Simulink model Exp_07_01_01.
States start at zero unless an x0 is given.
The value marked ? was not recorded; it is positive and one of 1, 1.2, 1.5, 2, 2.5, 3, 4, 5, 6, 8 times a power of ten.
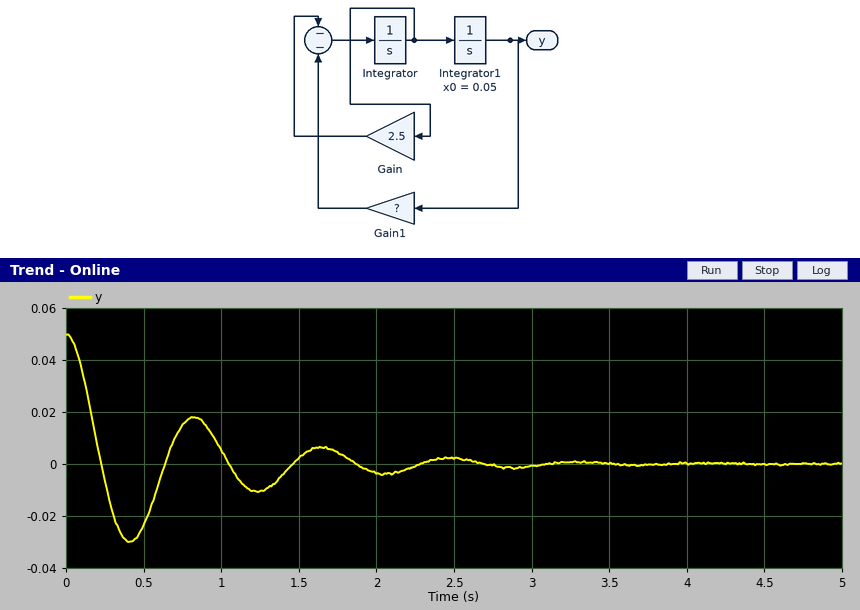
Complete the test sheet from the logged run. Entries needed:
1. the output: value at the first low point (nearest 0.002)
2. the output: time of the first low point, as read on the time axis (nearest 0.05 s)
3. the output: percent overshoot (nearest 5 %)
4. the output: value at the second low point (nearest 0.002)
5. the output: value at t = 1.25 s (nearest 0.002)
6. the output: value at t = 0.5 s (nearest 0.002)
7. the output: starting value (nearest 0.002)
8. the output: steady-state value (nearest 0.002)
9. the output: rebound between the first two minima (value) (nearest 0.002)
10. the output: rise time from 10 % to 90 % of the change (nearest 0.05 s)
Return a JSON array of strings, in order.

["-0.030", "0.40 s", "60 %", "-0.010", "-0.010", "-0.024", "0.050", "0.000", "0.018", "0.15 s"]
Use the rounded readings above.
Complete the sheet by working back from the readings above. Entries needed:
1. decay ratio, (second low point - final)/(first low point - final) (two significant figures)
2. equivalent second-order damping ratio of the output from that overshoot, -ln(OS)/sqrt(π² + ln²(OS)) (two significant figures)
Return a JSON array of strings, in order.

["0.33", "0.16"]
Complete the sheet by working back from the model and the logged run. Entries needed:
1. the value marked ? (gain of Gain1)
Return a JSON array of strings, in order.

["60"]
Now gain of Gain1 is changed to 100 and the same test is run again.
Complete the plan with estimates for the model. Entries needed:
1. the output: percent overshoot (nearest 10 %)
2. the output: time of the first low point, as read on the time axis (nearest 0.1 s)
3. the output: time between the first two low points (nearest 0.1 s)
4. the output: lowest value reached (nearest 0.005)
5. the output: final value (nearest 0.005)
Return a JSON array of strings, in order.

["70 %", "0.3 s", "0.6 s", "-0.035", "0.000"]
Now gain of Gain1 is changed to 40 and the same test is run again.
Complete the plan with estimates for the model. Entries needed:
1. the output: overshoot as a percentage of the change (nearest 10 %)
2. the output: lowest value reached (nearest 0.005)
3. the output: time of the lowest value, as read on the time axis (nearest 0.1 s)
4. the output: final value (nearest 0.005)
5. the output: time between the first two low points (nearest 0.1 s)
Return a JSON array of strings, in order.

["50 %", "-0.025", "0.5 s", "0.000", "1.0 s"]
